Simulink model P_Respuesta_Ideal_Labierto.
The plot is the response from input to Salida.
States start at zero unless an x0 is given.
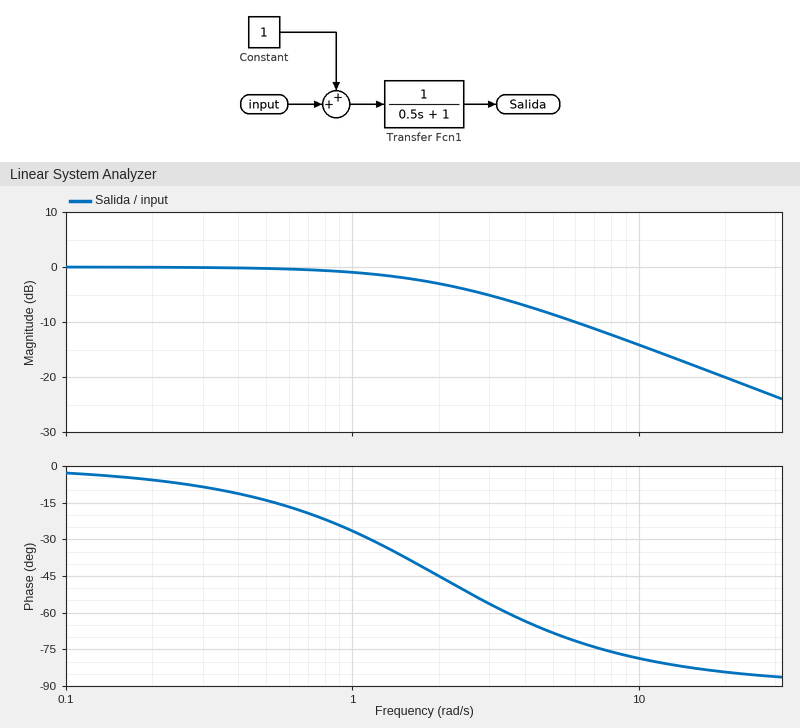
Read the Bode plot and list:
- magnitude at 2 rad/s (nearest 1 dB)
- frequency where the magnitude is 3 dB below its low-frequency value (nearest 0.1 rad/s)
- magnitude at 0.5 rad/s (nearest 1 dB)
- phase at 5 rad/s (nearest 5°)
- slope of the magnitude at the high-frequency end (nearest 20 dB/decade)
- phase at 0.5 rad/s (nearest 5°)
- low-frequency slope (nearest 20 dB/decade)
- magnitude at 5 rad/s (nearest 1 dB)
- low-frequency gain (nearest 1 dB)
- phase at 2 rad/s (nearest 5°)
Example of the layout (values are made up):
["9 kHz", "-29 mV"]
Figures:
["-3 dB", "2.0 rad/s", "0 dB", "-70°", "-20 dB/decade", "-15°", "0 dB/decade", "-9 dB", "0 dB", "-45°"]
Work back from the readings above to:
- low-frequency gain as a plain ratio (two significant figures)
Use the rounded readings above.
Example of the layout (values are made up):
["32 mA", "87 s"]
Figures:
["1.0"]
